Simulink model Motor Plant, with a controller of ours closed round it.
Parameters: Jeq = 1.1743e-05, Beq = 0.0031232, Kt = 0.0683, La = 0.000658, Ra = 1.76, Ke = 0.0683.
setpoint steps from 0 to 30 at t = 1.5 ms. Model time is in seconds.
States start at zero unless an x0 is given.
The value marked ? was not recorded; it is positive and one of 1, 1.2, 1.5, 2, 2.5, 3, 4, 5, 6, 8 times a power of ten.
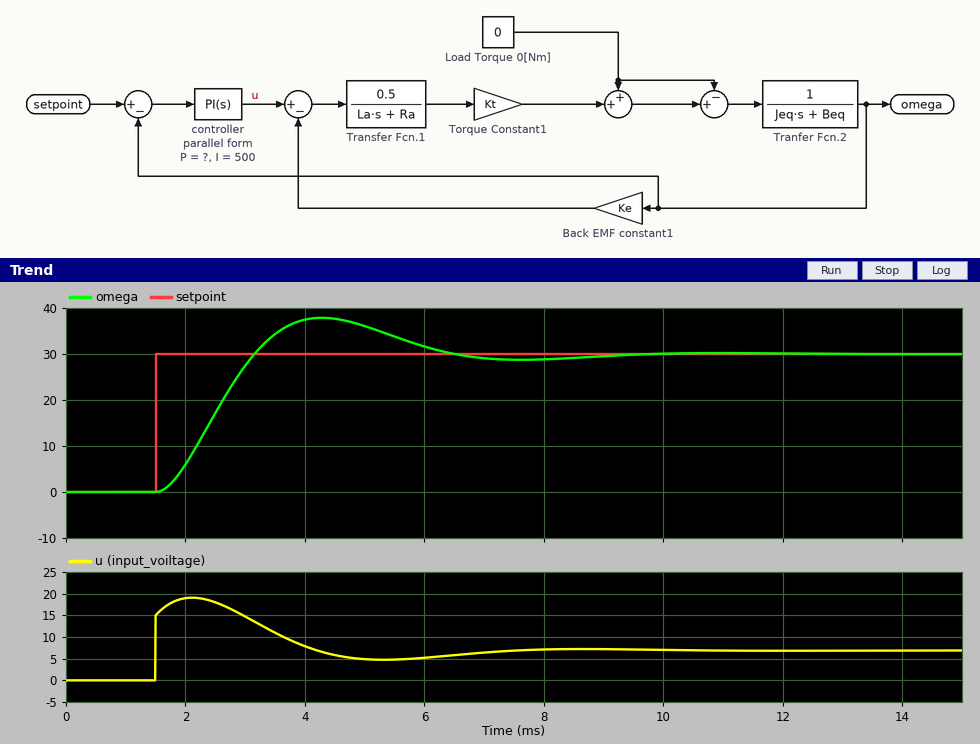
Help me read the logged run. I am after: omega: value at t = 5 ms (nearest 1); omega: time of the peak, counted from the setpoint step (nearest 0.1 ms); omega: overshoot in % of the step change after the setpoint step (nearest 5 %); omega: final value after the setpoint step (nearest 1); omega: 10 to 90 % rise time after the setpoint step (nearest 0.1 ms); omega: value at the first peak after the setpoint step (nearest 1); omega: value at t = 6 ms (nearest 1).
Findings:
36
2.8 ms
25 %
30
1.1 ms
38
32
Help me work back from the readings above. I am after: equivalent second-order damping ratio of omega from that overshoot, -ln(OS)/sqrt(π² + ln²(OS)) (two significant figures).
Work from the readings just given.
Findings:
0.40
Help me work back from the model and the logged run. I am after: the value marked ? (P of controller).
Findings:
0.5
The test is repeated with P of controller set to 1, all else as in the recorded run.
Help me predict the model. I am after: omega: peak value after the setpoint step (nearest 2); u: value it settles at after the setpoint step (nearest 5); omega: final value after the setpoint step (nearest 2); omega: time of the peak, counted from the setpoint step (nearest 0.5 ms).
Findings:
34
5
30
2.0 ms
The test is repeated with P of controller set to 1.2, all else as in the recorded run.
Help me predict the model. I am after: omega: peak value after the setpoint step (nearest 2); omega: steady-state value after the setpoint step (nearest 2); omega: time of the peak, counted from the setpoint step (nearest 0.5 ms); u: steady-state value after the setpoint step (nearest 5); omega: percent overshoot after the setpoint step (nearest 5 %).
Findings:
34
30
1.5 ms
5
15 %
